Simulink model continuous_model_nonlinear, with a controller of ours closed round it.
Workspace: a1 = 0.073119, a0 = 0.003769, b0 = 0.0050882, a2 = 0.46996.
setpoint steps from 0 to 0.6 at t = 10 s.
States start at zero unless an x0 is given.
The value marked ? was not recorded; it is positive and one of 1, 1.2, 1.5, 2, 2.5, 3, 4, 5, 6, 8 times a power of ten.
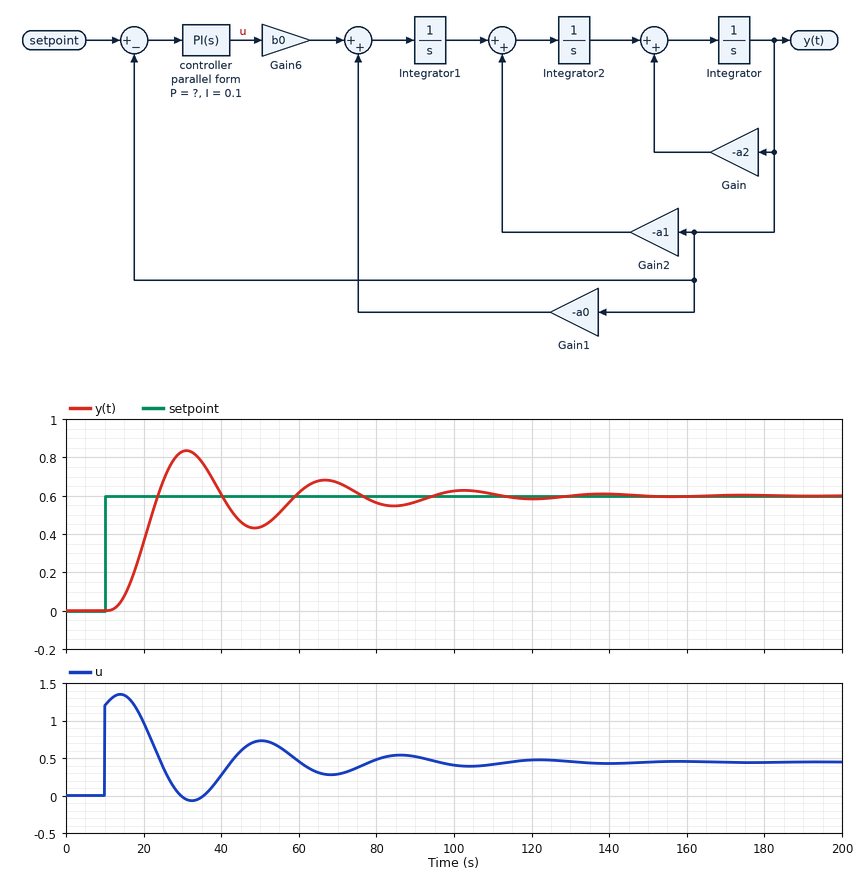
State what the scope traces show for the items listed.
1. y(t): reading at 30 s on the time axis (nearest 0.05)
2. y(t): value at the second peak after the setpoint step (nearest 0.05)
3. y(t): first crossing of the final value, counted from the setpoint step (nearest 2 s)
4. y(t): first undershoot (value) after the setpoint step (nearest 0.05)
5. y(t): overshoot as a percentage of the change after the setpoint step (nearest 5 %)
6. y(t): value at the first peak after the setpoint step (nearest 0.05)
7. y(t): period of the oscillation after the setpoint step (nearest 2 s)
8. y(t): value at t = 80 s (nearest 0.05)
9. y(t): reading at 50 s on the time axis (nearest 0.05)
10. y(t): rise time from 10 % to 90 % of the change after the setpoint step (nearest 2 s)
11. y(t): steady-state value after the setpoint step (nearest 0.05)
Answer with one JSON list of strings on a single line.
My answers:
["0.85", "0.70", "14 s", "0.45", "40 %", "0.85", "36 s", "0.55", "0.45", "8 s", "0.60"]
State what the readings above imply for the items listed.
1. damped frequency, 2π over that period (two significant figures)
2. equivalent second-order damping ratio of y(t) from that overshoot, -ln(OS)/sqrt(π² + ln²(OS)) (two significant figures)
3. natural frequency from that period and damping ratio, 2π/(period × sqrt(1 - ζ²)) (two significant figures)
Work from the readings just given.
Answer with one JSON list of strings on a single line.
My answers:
["0.17 rad/s", "0.28", "0.18 rad/s"]
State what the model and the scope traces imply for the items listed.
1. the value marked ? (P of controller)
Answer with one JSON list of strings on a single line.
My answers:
["2"]
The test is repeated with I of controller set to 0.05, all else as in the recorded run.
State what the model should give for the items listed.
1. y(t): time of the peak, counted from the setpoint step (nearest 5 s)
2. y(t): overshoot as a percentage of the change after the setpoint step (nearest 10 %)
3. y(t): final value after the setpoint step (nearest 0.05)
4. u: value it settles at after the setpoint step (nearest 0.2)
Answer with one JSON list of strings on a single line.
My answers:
["20 s", "20 %", "0.60", "0.4"]
